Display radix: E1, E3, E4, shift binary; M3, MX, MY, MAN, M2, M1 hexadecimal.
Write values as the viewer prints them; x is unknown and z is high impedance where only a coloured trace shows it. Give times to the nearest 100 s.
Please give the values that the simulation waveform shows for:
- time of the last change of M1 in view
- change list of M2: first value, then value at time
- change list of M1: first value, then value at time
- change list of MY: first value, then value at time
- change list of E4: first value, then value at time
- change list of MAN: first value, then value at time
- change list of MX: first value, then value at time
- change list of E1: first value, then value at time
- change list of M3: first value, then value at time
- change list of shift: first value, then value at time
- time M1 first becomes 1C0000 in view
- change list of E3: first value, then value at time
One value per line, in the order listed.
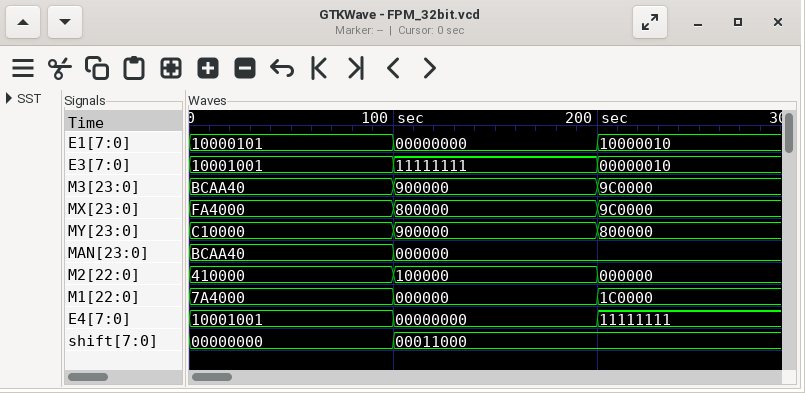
200 s
410000, 100000 at 100 s, 000000 at 200 s
7A4000, 000000 at 100 s, 1C0000 at 200 s
C10000, 900000 at 100 s, 800000 at 200 s
10001001, 00000000 at 100 s, 11111111 at 200 s
BCAA40, 000000 at 100 s
FA4000, 800000 at 100 s, 9C0000 at 200 s
10000101, 00000000 at 100 s, 10000010 at 200 s
BCAA40, 900000 at 100 s, 9C0000 at 200 s
00000000, 00011000 at 100 s
200 s
10001001, 11111111 at 100 s, 00000010 at 200 s
